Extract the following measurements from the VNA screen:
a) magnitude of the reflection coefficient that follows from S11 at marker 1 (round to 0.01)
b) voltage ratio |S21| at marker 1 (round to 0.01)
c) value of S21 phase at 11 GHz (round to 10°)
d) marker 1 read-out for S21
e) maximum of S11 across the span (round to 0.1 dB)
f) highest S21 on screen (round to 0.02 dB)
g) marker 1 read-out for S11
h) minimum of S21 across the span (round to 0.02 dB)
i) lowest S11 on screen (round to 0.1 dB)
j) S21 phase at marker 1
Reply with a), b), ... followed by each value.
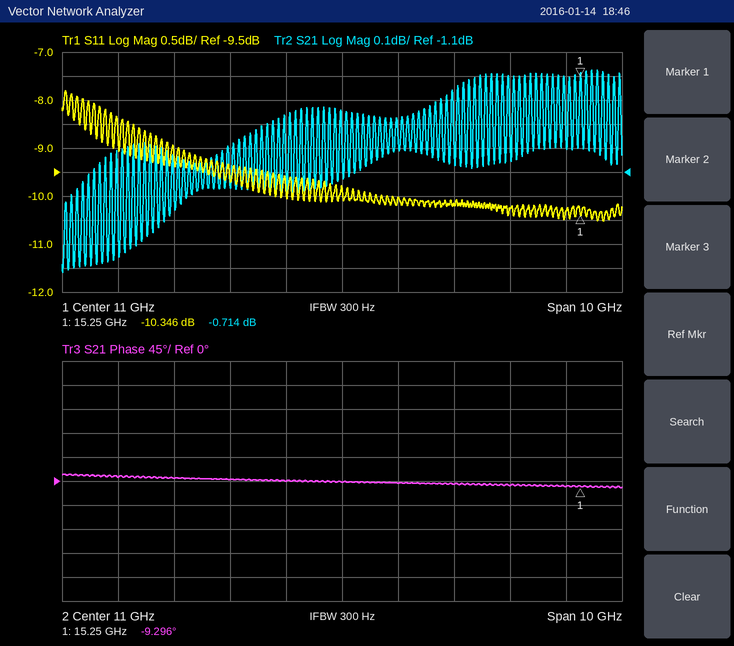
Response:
a) 0.30
b) 0.92
c) 0°
d) -0.714 dB
e) -7.8 dB
f) -0.68 dB
g) -10.346 dB
h) -1.52 dB
i) -10.5 dB
j) -9.296°
